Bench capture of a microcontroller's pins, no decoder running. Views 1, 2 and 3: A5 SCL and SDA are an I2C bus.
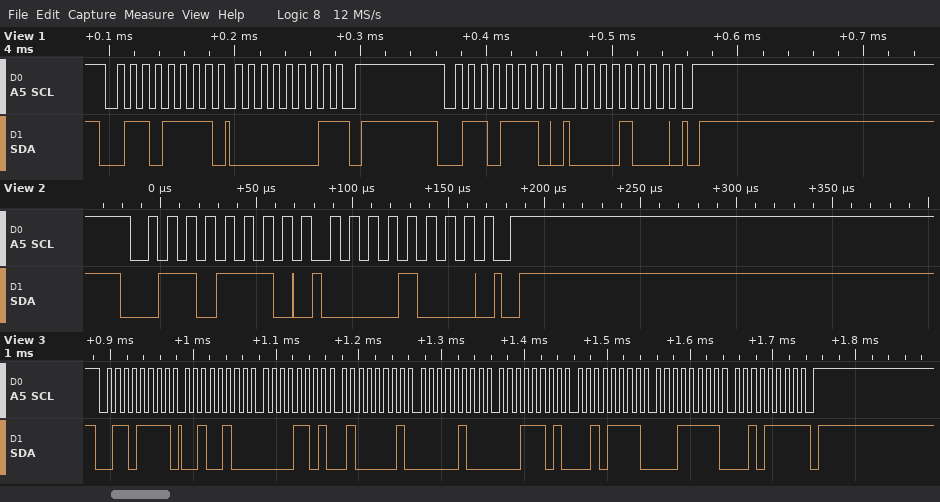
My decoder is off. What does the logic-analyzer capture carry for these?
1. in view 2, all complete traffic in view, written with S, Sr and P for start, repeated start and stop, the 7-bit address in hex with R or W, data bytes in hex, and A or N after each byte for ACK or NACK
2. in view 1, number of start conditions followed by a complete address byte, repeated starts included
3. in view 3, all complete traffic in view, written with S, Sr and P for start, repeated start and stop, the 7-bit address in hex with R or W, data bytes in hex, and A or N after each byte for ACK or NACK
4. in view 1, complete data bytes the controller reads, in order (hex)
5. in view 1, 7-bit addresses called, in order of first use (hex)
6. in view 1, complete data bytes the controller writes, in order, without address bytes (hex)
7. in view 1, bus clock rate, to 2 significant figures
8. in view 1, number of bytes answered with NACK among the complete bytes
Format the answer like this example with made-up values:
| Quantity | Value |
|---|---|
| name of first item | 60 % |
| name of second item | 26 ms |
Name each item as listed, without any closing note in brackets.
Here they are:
| Quantity | Value |
|---|---|
| in view 2, all complete traffic in view, written with S, Sr and P for start, repeated start and stop, the 7-bit address in hex with R or W, data bytes in hex, and A or N after each byte for ACK or NACK | S 37W A 08 A P |
| in view 1, number of start conditions followed by a complete address byte, repeated starts included | 2 |
| in view 3, all complete traffic in view, written with S, Sr and P for start, repeated start and stop, the 7-bit address in hex with R or W, data bytes in hex, and A or N after each byte for ACK or NACK | S 37R A 24 A 0D A 41 A 04 A 1D A 2F A 1F A 2F N P |
| in view 1, complete data bytes the controller reads, in order | 01 |
| in view 1, 7-bit addresses called, in order of first use | 0x37 |
| in view 1, complete data bytes the controller writes, in order, without address bytes | 08 |
| in view 1, bus clock rate, to 2 significant figures | 100 kHz |
| in view 1, number of bytes answered with NACK among the complete bytes | 1 |
